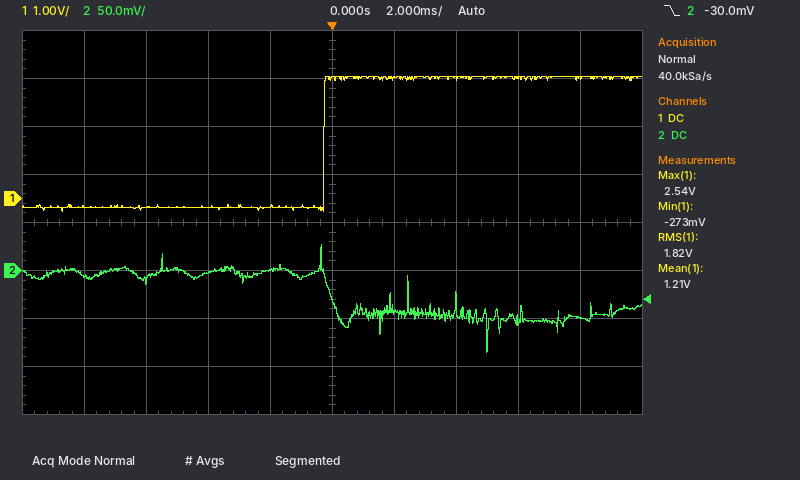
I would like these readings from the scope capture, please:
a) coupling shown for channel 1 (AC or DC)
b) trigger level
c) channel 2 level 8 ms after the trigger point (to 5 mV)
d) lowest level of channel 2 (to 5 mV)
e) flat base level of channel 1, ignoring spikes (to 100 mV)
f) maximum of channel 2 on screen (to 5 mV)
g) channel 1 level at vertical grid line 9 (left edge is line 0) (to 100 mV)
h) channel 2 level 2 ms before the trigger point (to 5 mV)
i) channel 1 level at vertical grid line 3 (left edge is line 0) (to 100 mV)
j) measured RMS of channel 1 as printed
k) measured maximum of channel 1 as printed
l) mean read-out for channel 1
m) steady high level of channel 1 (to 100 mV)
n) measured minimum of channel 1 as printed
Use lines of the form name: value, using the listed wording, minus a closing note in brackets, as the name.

coupling shown for channel 1: DC
trigger level: -30.0 mV
channel 2 level 8 ms after the trigger point: -50 mV
lowest level of channel 2: -85 mV
flat base level of channel 1, ignoring spikes: -200 mV
maximum of channel 2 on screen: 25 mV
channel 1 level at vertical grid line 9 (left edge is line 0): 2.5 V
channel 2 level 2 ms before the trigger point: 0 mV
channel 1 level at vertical grid line 3 (left edge is line 0): -200 mV
measured RMS of channel 1 as printed: 1.82 V
measured maximum of channel 1 as printed: 2.54 V
mean read-out for channel 1: 1.21 V
steady high level of channel 1: 2.5 V
measured minimum of channel 1 as printed: -273 mV
